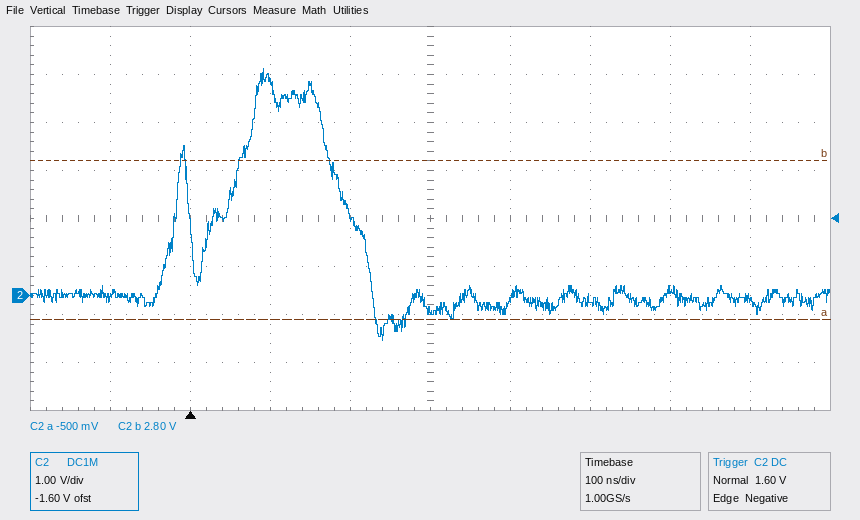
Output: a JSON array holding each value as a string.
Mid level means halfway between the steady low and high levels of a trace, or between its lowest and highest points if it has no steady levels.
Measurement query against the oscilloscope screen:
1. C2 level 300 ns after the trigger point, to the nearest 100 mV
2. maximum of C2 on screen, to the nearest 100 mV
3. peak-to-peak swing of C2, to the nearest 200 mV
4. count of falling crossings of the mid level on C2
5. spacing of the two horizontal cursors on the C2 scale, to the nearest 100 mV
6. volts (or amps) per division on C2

["-300 mV", "4.7 V", "5.6 V", "2", "3.3 V", "1 V"]
